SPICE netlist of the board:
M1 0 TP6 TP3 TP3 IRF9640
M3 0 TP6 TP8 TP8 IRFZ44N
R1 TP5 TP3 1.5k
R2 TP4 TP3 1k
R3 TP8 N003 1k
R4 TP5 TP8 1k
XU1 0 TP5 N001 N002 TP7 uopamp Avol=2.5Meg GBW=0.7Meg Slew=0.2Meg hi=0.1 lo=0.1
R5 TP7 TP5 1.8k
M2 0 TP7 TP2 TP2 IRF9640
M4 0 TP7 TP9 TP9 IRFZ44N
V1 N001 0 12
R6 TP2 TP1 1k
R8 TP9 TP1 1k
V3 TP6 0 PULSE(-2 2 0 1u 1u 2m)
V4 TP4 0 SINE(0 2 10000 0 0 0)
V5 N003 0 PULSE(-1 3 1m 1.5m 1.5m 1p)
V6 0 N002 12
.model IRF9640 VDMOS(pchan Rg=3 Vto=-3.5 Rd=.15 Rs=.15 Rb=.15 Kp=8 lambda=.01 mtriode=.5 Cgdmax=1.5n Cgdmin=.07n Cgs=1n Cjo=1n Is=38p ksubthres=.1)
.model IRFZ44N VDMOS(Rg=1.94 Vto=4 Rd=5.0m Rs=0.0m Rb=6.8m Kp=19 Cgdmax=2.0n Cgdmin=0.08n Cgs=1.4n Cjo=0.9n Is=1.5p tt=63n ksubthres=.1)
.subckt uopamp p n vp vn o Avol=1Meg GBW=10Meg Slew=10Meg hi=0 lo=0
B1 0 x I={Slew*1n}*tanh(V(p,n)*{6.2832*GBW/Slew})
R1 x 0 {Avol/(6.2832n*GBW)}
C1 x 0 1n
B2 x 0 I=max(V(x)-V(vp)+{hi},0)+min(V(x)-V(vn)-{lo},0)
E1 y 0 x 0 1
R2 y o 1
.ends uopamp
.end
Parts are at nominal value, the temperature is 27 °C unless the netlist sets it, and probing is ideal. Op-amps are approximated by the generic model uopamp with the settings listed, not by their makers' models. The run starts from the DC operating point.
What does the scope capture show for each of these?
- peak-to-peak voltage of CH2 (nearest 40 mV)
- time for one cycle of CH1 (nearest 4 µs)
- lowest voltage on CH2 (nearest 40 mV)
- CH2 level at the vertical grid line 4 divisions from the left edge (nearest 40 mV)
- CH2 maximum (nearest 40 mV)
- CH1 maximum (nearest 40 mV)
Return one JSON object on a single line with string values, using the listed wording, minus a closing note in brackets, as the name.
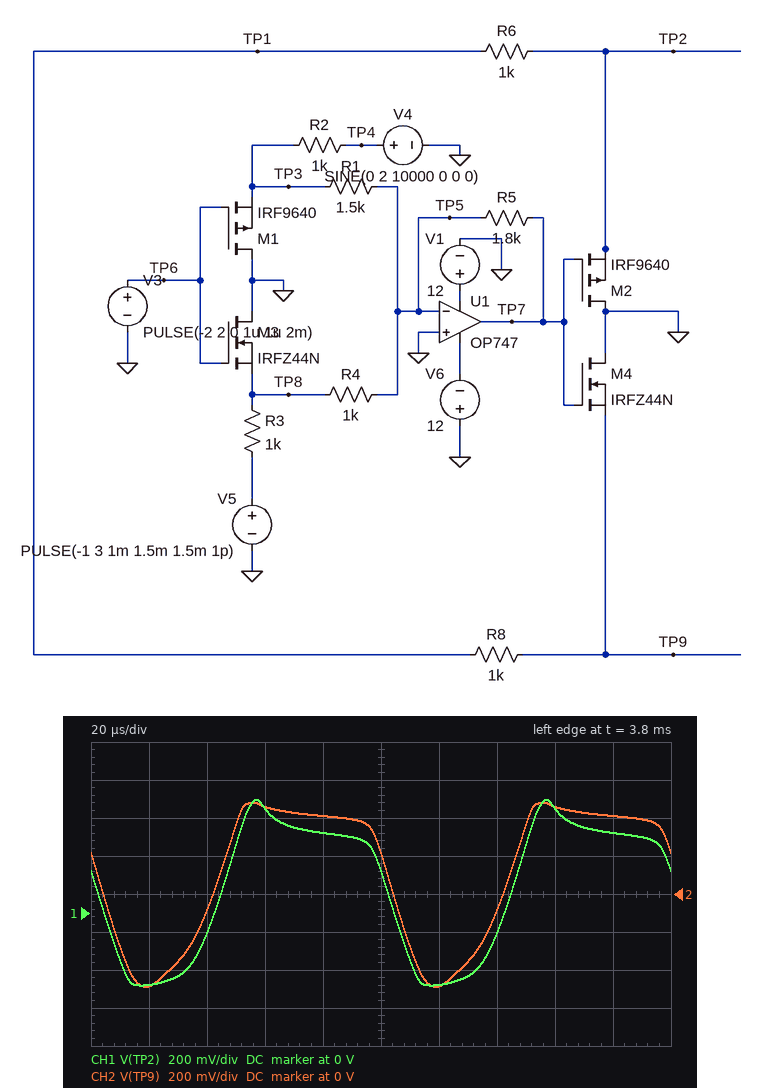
{"peak-to-peak voltage of CH2": "960 mV", "time for one cycle of CH1": "100 µs", "lowest voltage on CH2": "-480 mV", "CH2 level at the vertical grid line 4 divisions from the left edge": "400 mV", "CH2 maximum": "480 mV", "CH1 maximum": "600 mV"}
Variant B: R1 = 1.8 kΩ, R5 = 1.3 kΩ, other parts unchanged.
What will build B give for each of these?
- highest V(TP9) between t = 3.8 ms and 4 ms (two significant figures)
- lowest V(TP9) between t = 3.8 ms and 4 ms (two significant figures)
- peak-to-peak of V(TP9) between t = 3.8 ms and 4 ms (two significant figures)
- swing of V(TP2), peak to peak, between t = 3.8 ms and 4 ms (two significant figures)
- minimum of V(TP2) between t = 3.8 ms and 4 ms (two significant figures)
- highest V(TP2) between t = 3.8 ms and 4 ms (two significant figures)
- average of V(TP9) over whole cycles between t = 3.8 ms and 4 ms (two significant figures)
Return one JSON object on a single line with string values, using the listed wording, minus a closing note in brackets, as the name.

{"highest V(TP9) between t = 3.8 ms and 4 ms": "430 mV", "lowest V(TP9) between t = 3.8 ms and 4 ms": "-240 mV", "peak-to-peak of V(TP9) between t = 3.8 ms and 4 ms": "660 mV", "swing of V(TP2), peak to peak, between t = 3.8 ms and 4 ms": "670 mV", "minimum of V(TP2) between t = 3.8 ms and 4 ms": "-230 mV", "highest V(TP2) between t = 3.8 ms and 4 ms": "440 mV", "average of V(TP9) over whole cycles between t = 3.8 ms and 4 ms": "160 mV"}
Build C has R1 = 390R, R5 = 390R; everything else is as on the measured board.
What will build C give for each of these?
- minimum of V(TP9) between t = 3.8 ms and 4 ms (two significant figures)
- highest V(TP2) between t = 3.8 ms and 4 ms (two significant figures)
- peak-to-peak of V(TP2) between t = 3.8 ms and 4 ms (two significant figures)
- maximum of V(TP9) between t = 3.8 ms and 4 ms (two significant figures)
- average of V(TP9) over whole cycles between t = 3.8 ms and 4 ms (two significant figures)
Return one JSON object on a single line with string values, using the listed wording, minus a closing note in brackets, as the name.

{"minimum of V(TP9) between t = 3.8 ms and 4 ms": "-150 mV", "highest V(TP2) between t = 3.8 ms and 4 ms": "400 mV", "peak-to-peak of V(TP2) between t = 3.8 ms and 4 ms": "550 mV", "maximum of V(TP9) between t = 3.8 ms and 4 ms": "390 mV", "average of V(TP9) over whole cycles between t = 3.8 ms and 4 ms": "150 mV"}
